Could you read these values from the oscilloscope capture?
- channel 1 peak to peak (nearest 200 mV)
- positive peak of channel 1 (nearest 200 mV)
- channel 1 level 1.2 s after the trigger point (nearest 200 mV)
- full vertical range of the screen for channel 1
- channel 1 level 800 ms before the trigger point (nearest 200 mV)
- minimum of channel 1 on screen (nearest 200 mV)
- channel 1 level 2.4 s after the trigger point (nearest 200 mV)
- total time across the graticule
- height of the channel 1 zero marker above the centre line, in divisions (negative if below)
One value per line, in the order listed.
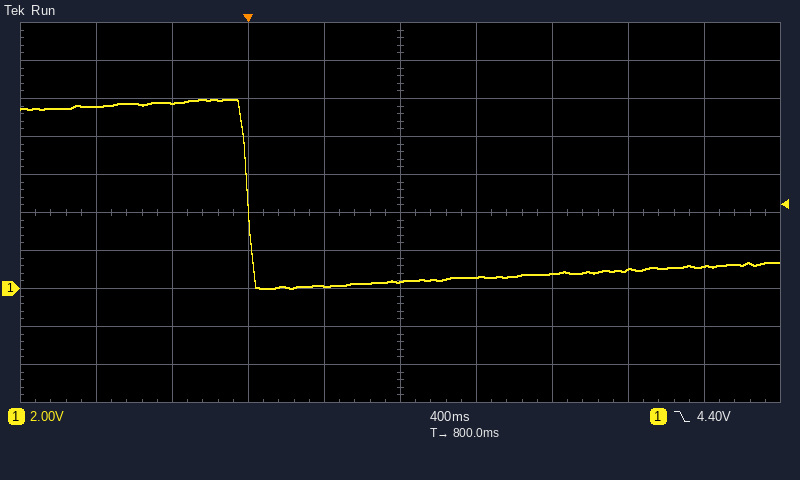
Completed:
10.0 V
10.0 V
600 mV
20 V
9.6 V
0.0 V
1.2 V
4 s
-2.0 div
